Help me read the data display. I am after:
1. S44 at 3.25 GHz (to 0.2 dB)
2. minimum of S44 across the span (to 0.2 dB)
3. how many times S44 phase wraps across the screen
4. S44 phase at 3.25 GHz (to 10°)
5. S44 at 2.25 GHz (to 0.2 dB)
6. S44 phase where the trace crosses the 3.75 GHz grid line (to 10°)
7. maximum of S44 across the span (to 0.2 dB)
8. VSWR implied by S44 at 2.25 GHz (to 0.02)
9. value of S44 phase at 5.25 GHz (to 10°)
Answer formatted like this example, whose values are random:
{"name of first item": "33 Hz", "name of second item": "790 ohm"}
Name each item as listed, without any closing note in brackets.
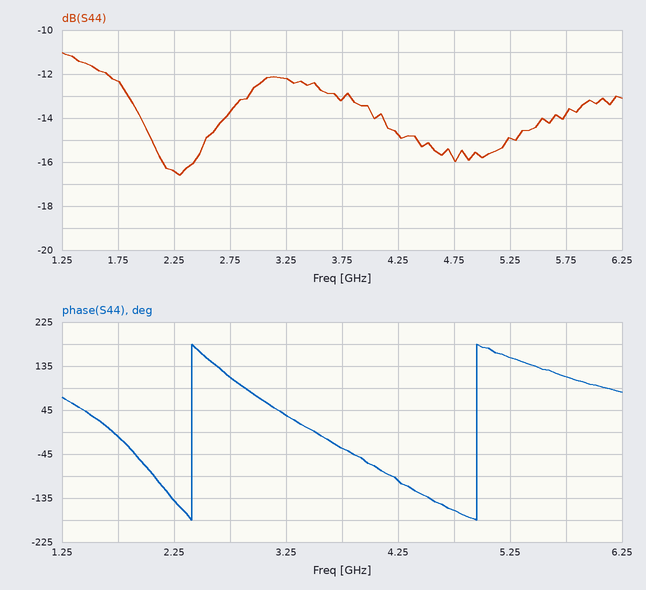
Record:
{"S44 at 3.25 GHz": "-12.2 dB", "minimum of S44 across the span": "-16.6 dB", "how many times S44 phase wraps across the screen": "2", "S44 phase at 3.25 GHz": "30°", "S44 at 2.25 GHz": "-16.4 dB", "S44 phase where the trace crosses the 3.75 GHz grid line": "-30°", "maximum of S44 across the span": "-11.0 dB", "VSWR implied by S44 at 2.25 GHz": "1.36", "value of S44 phase at 5.25 GHz": "150°"}
